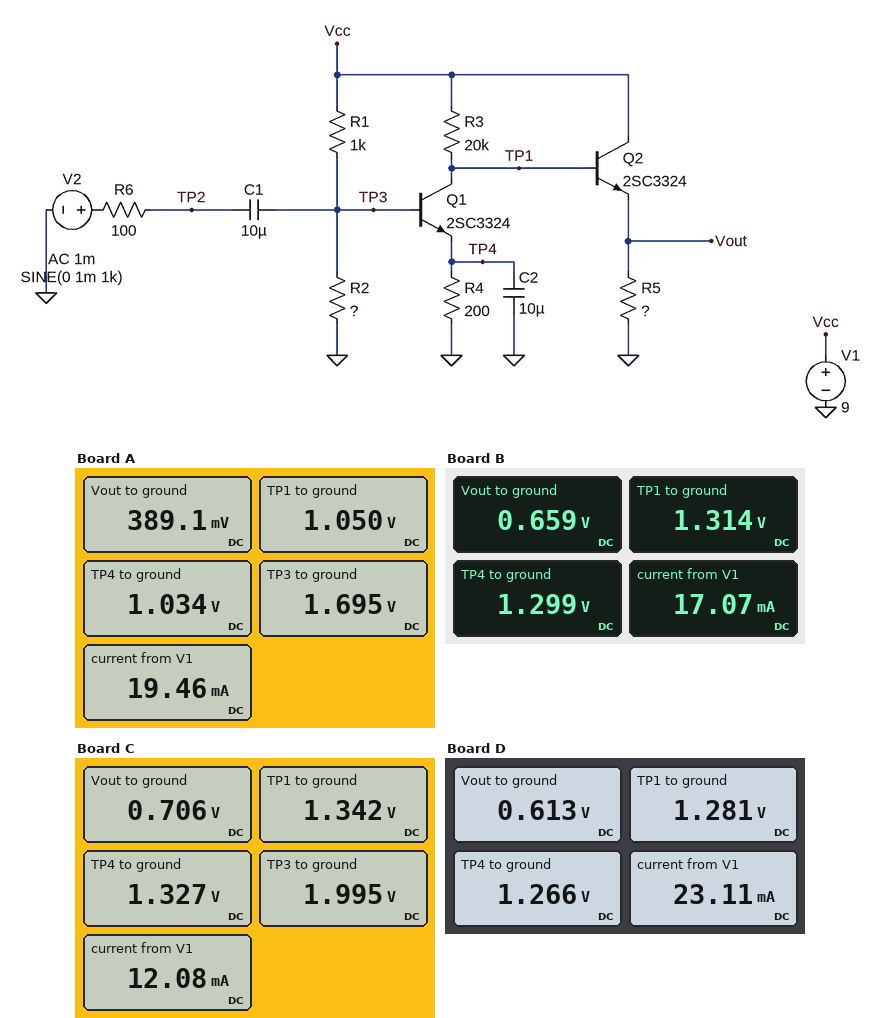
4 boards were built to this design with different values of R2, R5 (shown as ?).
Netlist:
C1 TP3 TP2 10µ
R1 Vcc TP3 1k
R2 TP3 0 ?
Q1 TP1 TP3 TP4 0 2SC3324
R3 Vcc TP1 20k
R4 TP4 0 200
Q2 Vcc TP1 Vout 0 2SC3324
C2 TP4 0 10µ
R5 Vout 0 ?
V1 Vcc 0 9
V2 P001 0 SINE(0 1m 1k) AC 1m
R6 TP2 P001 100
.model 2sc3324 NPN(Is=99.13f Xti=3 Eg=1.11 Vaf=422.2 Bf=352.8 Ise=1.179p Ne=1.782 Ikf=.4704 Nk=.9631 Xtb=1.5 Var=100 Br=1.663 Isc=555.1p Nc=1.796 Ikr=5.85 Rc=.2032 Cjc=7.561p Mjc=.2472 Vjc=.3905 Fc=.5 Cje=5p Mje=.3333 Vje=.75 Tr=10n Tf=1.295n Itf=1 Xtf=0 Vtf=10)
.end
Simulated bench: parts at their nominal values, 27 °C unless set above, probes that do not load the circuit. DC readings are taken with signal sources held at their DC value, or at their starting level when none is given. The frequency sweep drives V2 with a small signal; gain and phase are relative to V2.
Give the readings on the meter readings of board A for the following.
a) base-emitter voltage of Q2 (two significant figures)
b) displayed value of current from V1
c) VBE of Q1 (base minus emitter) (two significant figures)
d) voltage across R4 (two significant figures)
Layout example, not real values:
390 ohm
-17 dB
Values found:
660 mV
19.46 mA
660 mV
1.0 V
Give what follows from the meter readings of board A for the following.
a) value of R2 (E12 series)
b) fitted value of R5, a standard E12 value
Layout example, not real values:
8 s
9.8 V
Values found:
680 Ω
33 Ω
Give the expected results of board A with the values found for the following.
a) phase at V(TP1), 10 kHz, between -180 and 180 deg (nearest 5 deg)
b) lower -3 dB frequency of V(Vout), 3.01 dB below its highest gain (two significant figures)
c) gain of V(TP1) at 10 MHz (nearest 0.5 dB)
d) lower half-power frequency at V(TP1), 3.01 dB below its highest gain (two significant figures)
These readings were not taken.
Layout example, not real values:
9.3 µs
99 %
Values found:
-95 deg
40 Hz
-37.0 dB
40 Hz
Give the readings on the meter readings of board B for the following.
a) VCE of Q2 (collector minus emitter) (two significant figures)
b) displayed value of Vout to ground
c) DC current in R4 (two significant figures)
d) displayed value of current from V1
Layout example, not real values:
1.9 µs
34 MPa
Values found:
8.3 V
0.659 V
6.5 mA
17.07 mA
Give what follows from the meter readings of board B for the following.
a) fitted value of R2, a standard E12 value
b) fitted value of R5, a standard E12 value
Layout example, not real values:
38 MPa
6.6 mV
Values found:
2.2 kΩ
68 Ω
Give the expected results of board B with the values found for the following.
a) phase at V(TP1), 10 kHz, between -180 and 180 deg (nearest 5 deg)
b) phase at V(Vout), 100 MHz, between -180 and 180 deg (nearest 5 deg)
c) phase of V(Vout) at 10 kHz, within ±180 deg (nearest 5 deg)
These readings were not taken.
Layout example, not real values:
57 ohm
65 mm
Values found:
-90 deg
-30 deg
-90 deg
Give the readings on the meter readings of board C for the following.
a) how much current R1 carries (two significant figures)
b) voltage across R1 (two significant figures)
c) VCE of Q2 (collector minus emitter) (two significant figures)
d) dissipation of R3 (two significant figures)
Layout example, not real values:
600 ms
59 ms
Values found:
7.0 mA
7.0 V
8.3 V
2.9 mW
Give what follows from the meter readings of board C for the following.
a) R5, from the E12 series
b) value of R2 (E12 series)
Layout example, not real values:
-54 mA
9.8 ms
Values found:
150 Ω
2.7 kΩ
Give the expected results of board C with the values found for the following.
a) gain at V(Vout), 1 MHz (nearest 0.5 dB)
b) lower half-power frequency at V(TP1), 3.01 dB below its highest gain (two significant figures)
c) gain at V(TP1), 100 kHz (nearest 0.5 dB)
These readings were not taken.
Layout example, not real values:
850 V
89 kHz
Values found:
-56.0 dB
35 Hz
-56.5 dB
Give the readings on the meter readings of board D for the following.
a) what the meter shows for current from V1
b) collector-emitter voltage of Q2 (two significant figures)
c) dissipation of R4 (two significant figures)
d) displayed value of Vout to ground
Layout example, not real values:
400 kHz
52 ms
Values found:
23.11 mA
8.4 V
8.0 mW
0.613 V
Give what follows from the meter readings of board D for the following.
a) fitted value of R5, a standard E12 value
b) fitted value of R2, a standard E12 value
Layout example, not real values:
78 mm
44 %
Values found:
39 Ω
1.8 kΩ
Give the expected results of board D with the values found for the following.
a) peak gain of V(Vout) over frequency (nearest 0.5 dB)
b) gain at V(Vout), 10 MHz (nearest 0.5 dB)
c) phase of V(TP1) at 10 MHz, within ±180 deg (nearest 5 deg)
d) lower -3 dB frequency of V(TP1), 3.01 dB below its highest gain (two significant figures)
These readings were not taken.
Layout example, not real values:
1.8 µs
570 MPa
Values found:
-9.0 dB
-39.0 dB
40 deg
36 Hz
